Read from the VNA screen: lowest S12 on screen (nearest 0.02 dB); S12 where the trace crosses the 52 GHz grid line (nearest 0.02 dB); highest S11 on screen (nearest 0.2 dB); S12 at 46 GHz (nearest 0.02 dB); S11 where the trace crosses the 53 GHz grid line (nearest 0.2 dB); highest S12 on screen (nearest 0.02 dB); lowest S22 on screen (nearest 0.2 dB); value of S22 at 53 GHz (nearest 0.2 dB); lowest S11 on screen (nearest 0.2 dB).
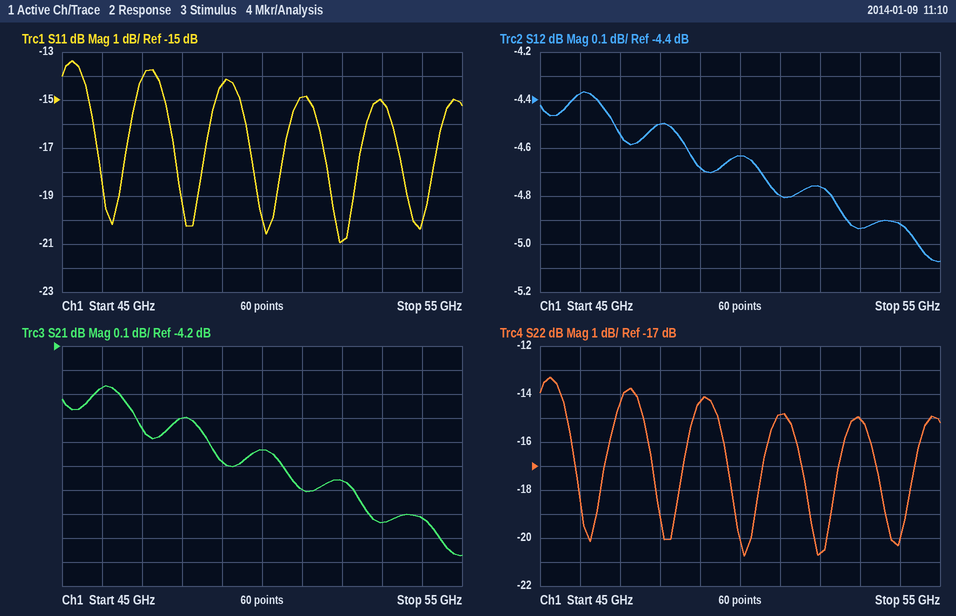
-5.08 dB
-4.76 dB
-13.4 dB
-4.38 dB
-15.0 dB
-4.36 dB
-20.8 dB
-15.0 dB
-21.0 dB
